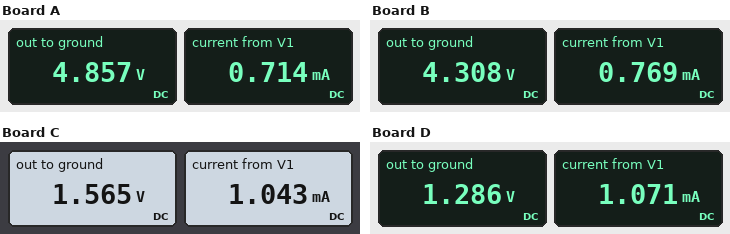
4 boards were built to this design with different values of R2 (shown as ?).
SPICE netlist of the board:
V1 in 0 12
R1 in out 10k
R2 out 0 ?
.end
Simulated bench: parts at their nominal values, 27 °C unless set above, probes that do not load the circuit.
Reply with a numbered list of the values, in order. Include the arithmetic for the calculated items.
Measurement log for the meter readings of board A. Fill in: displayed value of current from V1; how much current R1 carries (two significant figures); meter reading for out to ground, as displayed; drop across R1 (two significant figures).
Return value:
1. 0.714 mA
2. (12 V - 4.857 V) / 10 kΩ = 710 µA
3. 4.857 V
4. 12 V - 4.857 V = 7.1 V
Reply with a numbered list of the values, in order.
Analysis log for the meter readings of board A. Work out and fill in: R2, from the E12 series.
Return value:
1. 6.8 kΩ
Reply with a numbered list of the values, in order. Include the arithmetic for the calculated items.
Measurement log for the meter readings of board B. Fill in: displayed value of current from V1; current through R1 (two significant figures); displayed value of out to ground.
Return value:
1. 0.769 mA
2. (12 V - 4.308 V) / 10 kΩ = 770 µA
3. 4.308 V
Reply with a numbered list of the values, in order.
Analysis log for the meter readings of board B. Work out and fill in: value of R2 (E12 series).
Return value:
1. 5.6 kΩ
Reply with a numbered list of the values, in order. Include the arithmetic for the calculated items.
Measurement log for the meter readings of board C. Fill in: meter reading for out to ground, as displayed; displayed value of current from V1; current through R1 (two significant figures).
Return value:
1. 1.565 V
2. 1.043 mA
3. (12 V - 1.565 V) / 10 kΩ = 1.0 mA
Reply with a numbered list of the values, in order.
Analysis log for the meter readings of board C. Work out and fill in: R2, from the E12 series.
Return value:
1. 1.5 kΩ
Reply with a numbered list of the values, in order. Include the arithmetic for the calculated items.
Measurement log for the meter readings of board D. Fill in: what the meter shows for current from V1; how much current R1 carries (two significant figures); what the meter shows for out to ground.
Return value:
1. 1.071 mA
2. (12 V - 1.286 V) / 10 kΩ = 1.1 mA
3. 1.286 V
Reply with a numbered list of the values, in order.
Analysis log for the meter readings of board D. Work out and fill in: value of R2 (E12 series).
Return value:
1. 1.2 kΩ
